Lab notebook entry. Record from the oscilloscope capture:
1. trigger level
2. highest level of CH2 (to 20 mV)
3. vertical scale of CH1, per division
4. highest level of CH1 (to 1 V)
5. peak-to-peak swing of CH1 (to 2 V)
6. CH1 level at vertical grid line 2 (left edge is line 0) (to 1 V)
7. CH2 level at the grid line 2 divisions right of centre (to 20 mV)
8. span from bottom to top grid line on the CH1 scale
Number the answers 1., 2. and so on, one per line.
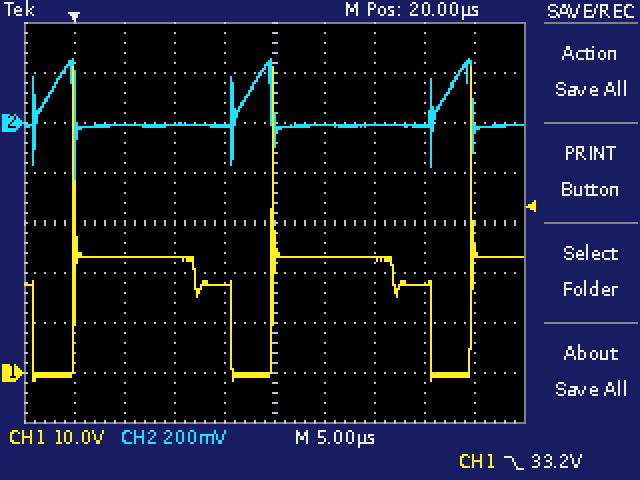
1. 33.2 V
2. 260 mV
3. 10 V
4. 61 V
5. 62 V
6. 23 V
7. 0 mV
8. 80 V
